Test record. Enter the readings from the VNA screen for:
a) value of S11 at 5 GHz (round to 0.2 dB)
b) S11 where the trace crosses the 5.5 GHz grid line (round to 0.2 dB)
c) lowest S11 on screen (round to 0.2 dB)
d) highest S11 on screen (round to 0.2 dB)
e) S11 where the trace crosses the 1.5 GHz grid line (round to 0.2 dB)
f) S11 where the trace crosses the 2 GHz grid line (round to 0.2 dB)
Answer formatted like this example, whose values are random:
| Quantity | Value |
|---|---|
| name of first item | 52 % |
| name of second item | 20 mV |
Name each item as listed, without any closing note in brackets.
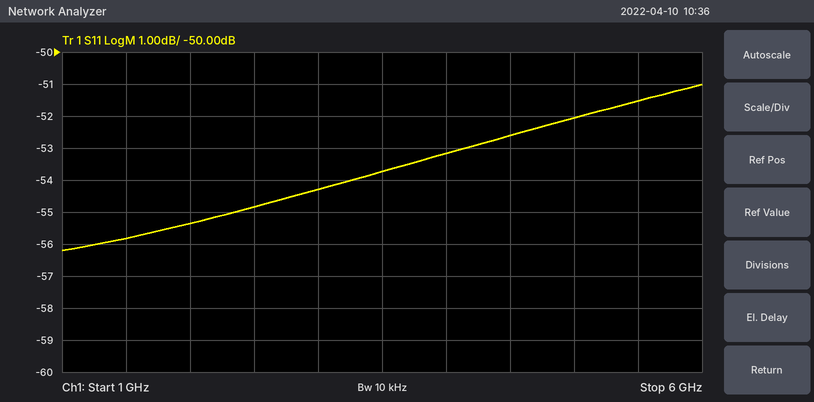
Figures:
| Quantity | Value |
|---|---|
| value of S11 at 5 GHz | -52.0 dB |
| S11 where the trace crosses the 5.5 GHz grid line | -51.6 dB |
| lowest S11 on screen | -56.2 dB |
| highest S11 on screen | -51.0 dB |
| S11 where the trace crosses the 1.5 GHz grid line | -55.8 dB |
| S11 where the trace crosses the 2 GHz grid line | -55.4 dB |
